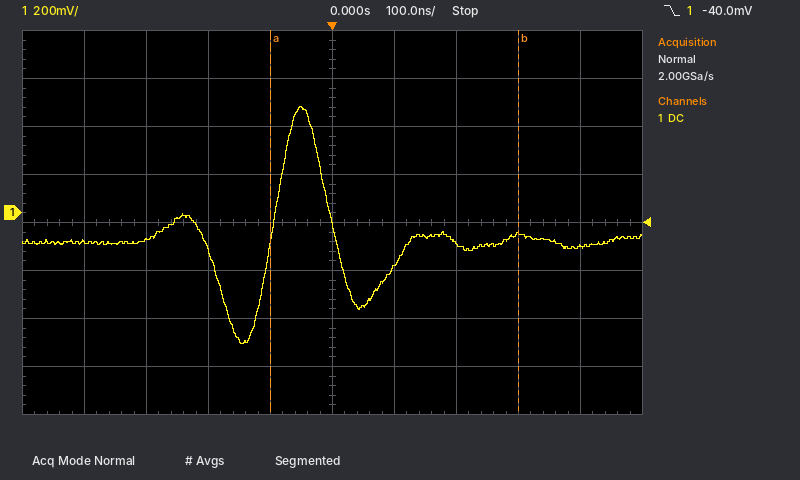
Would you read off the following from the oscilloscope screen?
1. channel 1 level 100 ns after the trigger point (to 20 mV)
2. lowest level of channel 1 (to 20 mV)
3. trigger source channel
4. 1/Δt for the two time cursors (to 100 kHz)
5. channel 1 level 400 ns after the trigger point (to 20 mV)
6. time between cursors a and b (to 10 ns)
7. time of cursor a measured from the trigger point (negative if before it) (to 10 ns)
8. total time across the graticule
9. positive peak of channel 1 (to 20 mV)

-220 mV
-540 mV
channel 1
2.5 MHz
-140 mV
400 ns
-100 ns
1 µs
440 mV
